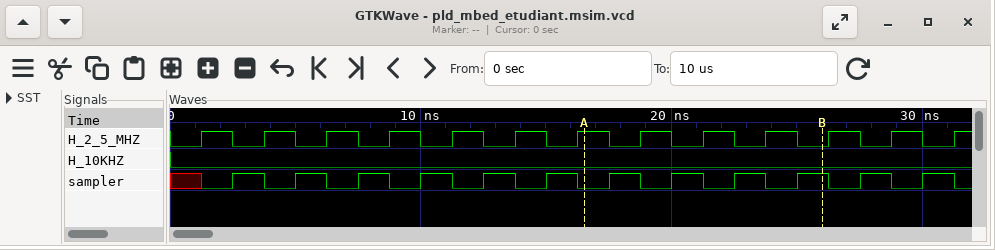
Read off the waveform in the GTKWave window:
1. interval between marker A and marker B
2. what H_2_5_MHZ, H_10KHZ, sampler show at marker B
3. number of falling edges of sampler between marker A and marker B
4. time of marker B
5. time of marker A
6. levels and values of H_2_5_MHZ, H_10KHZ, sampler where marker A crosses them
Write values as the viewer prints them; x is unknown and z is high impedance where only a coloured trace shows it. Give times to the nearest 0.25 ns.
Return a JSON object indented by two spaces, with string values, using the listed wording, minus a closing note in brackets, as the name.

{
  "interval between marker A and marker B": "9.5 ns",
  "what H_2_5_MHZ, H_10KHZ, sampler show at marker B": "H_2_5_MHZ=0, H_10KHZ=0, sampler=1",
  "number of falling edges of sampler between marker A and marker B": "3",
  "time of marker B": "26 ns",
  "time of marker A": "16.5 ns",
  "levels and values of H_2_5_MHZ, H_10KHZ, sampler where marker A crosses them": "H_2_5_MHZ=1, H_10KHZ=0, sampler=0"
}
